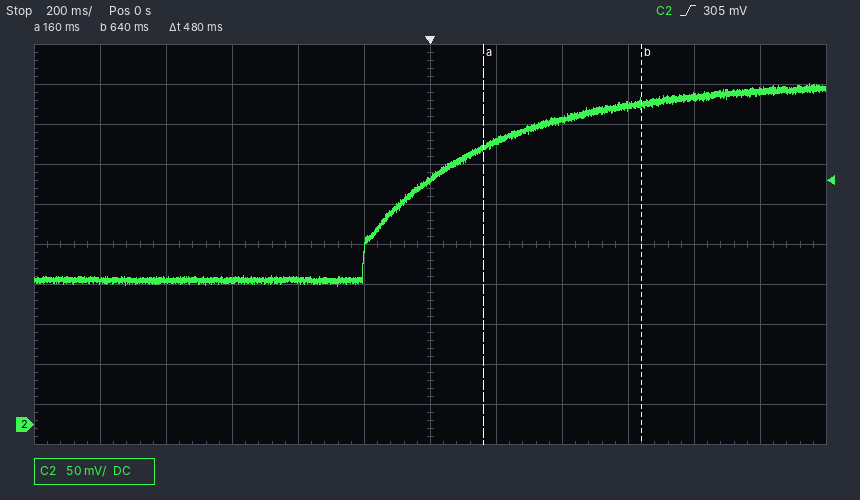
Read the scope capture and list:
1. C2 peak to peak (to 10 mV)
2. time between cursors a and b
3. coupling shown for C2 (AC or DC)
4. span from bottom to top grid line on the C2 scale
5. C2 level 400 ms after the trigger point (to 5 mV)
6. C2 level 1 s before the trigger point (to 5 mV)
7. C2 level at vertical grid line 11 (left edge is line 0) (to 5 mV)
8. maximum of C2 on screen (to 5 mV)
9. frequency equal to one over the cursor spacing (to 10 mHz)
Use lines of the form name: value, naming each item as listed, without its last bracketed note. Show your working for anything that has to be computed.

C2 peak to peak: 250 mV
time between cursors a and b: 480 ms
coupling shown for C2: DC
span from bottom to top grid line on the C2 scale: 500 mV
C2 level 400 ms after the trigger point: 380 mV
C2 level 1 s before the trigger point: 180 mV
C2 level at vertical grid line 11 (left edge is line 0): 415 mV
maximum of C2 on screen: 425 mV
frequency equal to one over the cursor spacing: 1 / 480 ms ≈ 2.08 Hz
